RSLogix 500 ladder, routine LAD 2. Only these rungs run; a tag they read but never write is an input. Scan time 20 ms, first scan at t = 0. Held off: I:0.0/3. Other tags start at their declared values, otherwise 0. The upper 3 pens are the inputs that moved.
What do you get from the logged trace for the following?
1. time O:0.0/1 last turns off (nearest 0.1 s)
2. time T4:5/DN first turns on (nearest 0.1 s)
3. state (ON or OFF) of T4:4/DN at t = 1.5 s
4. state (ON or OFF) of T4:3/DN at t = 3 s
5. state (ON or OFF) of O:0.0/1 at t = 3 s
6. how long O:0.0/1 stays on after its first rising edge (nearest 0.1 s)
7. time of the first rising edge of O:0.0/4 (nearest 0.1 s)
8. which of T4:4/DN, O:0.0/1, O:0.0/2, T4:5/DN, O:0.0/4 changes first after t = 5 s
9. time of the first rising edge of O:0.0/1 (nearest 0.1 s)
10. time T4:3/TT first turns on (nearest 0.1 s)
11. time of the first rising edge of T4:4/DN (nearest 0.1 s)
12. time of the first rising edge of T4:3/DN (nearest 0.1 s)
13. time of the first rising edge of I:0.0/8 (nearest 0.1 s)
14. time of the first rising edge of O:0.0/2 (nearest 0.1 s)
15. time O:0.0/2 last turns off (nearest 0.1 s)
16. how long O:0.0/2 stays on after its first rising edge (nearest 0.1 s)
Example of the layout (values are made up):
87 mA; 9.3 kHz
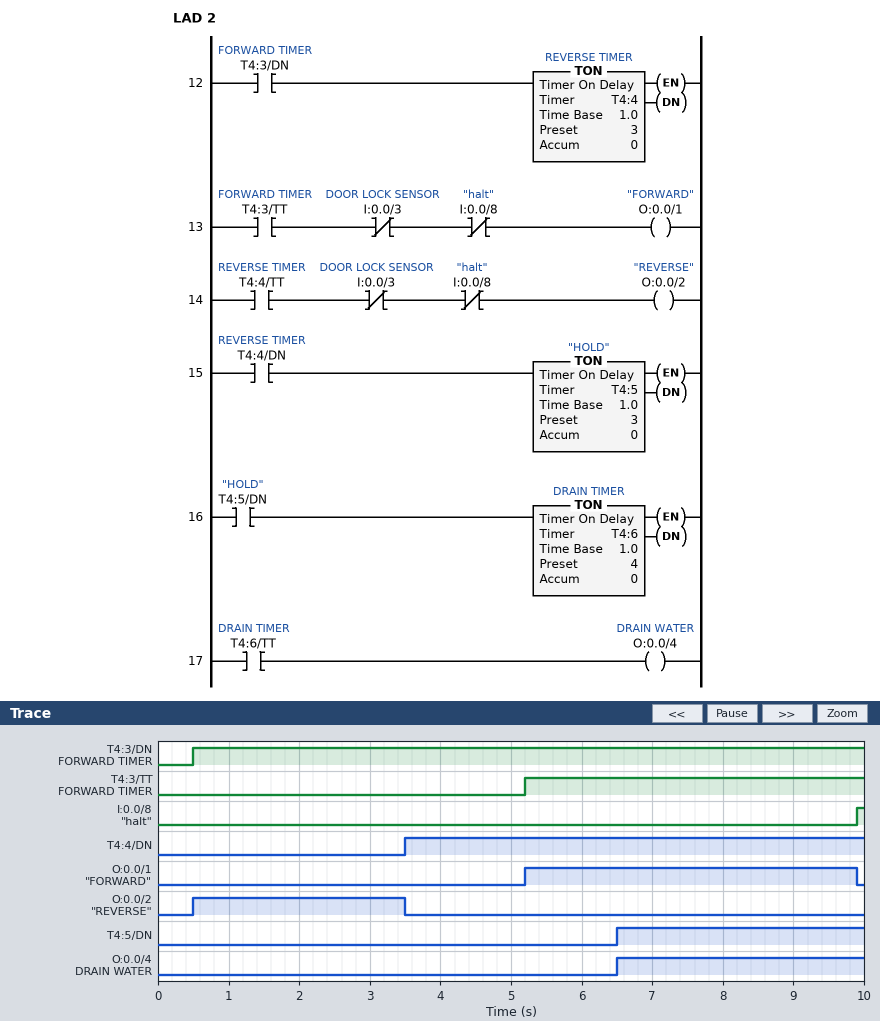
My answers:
9.9 s; 6.5 s; OFF; ON; OFF; 4.7 s; 6.5 s; O:0.0/1; 5.2 s; 5.2 s; 3.5 s; 0.5 s; 9.9 s; 0.5 s; 3.5 s; 3.0 s
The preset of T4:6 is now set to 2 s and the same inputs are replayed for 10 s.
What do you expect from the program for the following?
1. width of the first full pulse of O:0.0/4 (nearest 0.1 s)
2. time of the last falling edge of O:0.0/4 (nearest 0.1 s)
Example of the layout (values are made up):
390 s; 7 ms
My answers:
2.0 s; 8.5 s
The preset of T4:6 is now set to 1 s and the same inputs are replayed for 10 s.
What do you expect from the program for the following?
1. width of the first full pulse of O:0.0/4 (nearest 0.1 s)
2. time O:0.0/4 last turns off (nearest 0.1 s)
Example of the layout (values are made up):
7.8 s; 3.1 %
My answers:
1.0 s; 7.5 s
